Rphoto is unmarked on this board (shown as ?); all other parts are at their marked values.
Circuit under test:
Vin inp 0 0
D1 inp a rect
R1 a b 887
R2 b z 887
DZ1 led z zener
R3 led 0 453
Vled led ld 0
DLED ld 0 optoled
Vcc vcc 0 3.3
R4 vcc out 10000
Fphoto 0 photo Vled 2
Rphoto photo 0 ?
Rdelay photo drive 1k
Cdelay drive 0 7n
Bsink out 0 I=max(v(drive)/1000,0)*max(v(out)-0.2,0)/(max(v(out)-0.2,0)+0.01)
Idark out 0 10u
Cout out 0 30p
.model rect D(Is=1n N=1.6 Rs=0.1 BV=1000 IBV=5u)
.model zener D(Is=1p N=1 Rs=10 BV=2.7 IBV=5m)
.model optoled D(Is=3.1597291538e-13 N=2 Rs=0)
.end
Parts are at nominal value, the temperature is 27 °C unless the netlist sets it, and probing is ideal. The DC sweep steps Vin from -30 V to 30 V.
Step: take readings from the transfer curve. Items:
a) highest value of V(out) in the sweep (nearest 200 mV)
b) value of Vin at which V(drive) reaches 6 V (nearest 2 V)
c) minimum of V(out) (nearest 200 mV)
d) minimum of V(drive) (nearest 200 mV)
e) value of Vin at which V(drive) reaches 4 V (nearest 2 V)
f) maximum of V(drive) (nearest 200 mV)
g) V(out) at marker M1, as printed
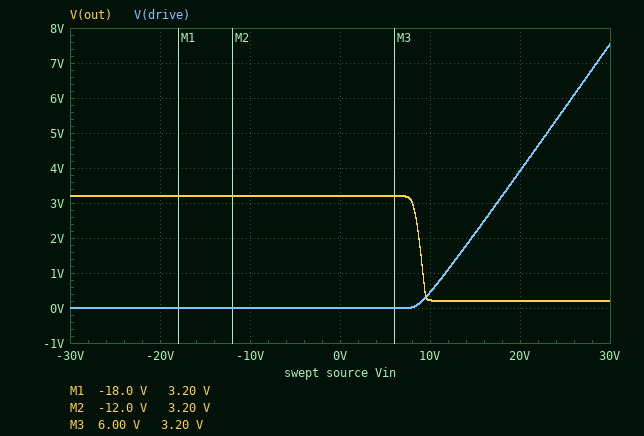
3.2 V
26 V
200 mV
0 V
20 V
7.6 V
3.20 V
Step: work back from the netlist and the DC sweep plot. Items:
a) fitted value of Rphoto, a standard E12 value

330 Ω
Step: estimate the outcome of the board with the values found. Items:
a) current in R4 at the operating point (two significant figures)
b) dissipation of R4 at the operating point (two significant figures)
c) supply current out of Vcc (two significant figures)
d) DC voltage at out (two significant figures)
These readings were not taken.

10 µA
1.0 µW
10 µA
3.2 V
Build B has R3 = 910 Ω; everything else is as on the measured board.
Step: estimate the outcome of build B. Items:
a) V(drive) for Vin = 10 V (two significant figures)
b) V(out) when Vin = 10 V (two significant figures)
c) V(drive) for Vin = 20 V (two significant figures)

1.2 V
200 mV
4.8 V
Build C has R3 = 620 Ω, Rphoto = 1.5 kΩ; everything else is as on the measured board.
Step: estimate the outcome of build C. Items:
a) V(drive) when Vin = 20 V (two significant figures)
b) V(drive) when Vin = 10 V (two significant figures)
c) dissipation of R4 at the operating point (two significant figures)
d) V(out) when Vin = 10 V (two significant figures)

20 V
3.8 V
1.0 µW
200 mV
